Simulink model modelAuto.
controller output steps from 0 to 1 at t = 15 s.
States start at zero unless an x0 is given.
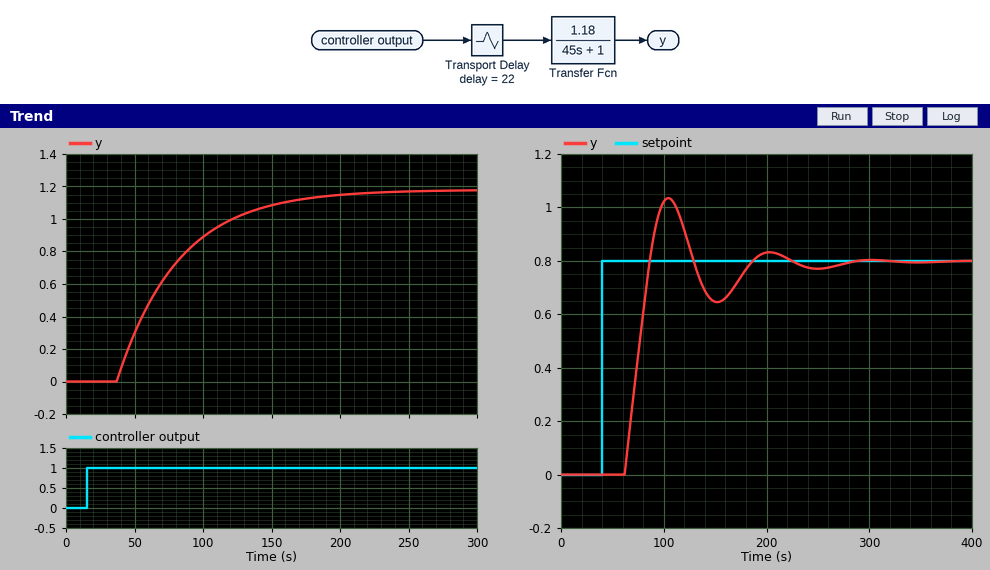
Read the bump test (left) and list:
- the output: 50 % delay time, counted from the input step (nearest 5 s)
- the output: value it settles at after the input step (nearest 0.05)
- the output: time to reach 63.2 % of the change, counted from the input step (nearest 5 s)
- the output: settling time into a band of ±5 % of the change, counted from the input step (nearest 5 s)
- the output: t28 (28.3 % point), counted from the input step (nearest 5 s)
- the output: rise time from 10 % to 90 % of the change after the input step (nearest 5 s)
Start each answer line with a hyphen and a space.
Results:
- 55 s
- 1.20
- 65 s
- 155 s
- 35 s
- 100 s
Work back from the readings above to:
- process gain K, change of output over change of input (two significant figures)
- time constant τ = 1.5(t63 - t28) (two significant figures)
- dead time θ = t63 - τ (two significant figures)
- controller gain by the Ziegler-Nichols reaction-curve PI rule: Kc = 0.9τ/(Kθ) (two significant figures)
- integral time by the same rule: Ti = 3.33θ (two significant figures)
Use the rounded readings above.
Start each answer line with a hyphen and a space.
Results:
- 1.2
- 45 s
- 20 s
- 1.7
- 67 s
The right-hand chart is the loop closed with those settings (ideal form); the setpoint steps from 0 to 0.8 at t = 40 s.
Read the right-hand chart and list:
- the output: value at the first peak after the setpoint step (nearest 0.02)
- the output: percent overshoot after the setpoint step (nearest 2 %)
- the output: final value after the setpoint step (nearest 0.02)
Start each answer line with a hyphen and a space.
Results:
- 1.04
- 30 %
- 0.80
